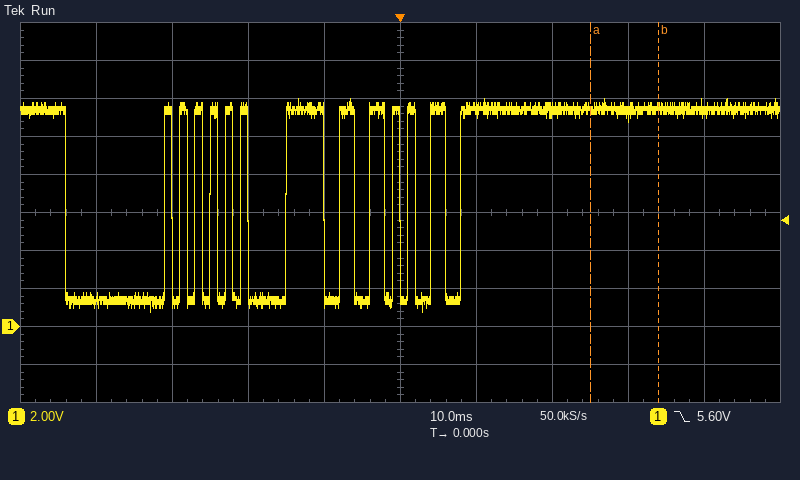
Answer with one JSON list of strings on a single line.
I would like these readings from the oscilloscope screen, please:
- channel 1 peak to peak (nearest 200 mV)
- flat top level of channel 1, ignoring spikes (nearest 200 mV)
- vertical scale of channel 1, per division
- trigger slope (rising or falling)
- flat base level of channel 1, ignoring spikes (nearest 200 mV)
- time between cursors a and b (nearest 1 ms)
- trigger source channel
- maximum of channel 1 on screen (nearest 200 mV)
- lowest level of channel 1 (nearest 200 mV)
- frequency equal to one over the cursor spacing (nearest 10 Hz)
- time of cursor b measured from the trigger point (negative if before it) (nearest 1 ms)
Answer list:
["11.2 V", "11.4 V", "2 V", "falling", "1.4 V", "9 ms", "channel 1", "12.0 V", "800 mV", "110 Hz", "+34 ms"]
